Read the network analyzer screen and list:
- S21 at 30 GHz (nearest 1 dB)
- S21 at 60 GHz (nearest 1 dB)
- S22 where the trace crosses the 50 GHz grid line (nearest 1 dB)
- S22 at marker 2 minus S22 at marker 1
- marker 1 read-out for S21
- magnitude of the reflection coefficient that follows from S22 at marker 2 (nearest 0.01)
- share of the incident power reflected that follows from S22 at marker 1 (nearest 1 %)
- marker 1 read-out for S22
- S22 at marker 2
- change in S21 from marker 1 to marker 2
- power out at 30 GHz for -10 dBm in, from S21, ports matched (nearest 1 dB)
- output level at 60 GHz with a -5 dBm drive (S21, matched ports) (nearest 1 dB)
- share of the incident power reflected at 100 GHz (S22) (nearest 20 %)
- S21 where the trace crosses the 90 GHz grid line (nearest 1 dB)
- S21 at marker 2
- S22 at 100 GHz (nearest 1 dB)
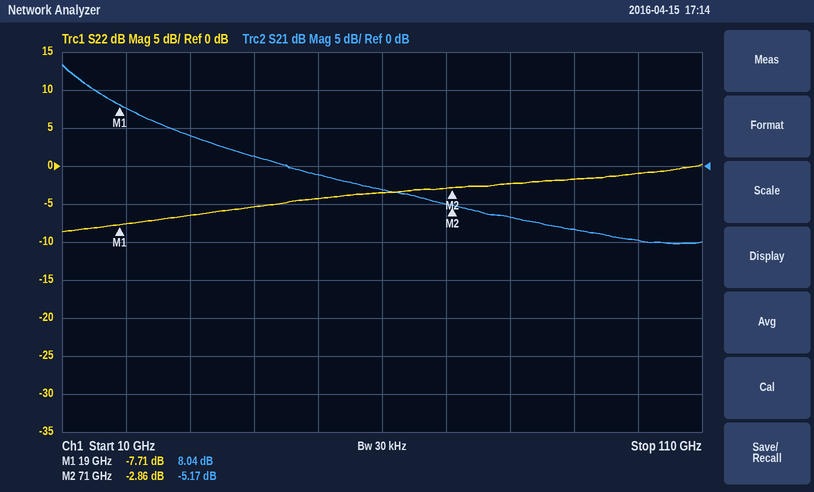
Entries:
4 dB
-3 dB
-4 dB
4.85 dB
8.04 dB
0.72
17 %
-7.71 dB
-2.86 dB
-13.21 dB
-6 dBm
-8 dBm
80 %
-8 dB
-5.17 dB
-1 dB
